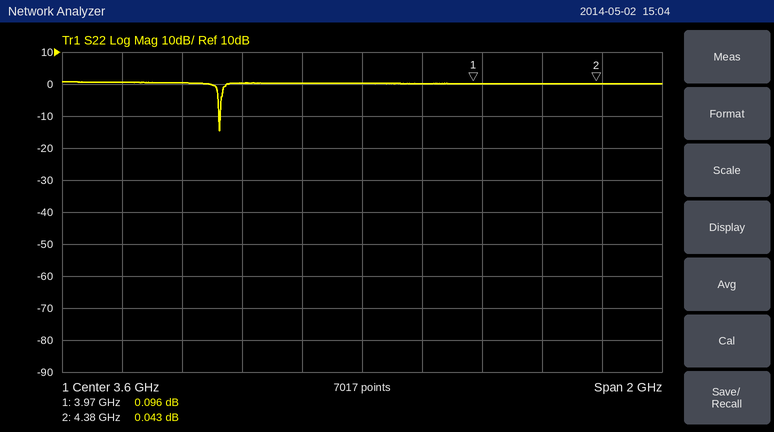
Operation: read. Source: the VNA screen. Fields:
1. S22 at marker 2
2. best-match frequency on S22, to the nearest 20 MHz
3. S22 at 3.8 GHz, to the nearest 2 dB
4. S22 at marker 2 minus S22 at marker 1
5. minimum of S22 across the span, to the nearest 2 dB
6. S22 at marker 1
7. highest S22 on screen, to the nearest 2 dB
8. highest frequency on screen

0.043 dB
3.12 GHz
0 dB
-0.053 dB
-14 dB
0.096 dB
0 dB
4.6 GHz
